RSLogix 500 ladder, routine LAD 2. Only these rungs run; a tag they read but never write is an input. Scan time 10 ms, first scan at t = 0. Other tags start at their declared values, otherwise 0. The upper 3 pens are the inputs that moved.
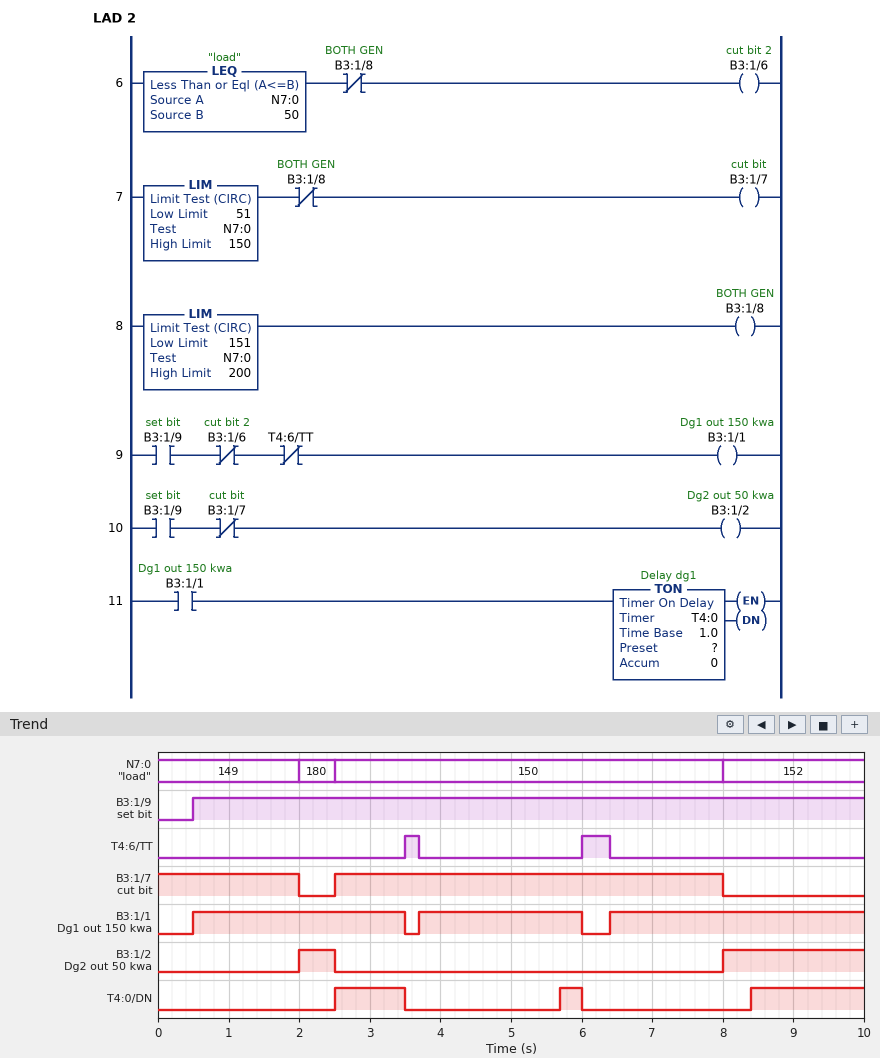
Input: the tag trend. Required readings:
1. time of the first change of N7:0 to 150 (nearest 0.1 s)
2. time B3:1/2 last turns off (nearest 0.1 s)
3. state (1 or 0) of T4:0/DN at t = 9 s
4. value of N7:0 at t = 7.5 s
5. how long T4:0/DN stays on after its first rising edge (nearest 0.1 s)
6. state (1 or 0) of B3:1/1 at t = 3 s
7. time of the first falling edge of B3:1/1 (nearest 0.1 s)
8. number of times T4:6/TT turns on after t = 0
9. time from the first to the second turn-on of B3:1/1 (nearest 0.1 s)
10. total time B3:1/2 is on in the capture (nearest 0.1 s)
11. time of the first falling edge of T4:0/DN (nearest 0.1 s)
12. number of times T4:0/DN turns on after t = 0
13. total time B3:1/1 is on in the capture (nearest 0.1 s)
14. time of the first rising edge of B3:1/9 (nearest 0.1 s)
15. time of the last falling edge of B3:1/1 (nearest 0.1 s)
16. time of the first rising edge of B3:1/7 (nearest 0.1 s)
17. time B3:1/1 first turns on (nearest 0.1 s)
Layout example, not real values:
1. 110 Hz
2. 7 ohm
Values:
1. 2.5 s
2. 2.5 s
3. 1
4. 150
5. 1.0 s
6. 1
7. 3.5 s
8. 2
9. 3.2 s
10. 2.5 s
11. 3.5 s
12. 3
13. 8.9 s
14. 0.5 s
15. 6.0 s
16. 2.5 s
17. 0.5 s
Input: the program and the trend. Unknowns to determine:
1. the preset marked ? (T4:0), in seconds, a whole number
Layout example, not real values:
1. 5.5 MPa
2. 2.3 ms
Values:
1. 2 s
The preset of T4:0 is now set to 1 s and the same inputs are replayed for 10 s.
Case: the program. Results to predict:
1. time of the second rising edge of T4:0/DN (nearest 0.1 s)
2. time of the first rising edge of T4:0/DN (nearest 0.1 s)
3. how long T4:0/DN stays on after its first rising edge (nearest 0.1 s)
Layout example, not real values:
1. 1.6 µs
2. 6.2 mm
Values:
1. 4.7 s
2. 1.5 s
3. 2.0 s
